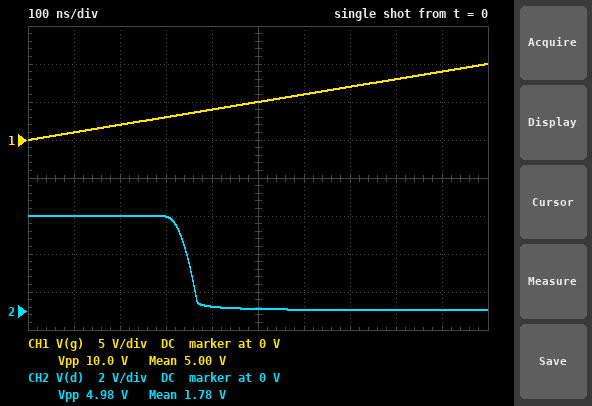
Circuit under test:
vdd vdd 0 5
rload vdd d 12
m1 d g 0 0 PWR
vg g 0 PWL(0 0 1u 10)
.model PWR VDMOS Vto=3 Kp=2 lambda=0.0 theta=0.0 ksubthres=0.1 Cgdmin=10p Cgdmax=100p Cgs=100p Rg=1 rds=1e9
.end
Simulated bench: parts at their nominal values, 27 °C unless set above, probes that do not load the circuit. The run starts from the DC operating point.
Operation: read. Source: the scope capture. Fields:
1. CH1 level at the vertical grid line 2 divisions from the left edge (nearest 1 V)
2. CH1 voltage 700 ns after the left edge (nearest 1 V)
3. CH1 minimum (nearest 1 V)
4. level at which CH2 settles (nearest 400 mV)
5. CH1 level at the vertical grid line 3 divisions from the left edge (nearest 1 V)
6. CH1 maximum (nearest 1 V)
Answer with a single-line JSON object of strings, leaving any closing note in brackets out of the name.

{"CH1 level at the vertical grid line 2 divisions from the left edge": "2 V", "CH1 voltage 700 ns after the left edge": "7 V", "CH1 minimum": "0 V", "level at which CH2 settles": "0 V", "CH1 level at the vertical grid line 3 divisions from the left edge": "3 V", "CH1 maximum": "10 V"}
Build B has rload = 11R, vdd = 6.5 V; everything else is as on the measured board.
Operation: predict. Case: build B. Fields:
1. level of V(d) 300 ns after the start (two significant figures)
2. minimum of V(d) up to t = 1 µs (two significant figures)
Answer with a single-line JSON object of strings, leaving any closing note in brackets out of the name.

{"level of V(d) 300 ns after the start": "6.5 V", "minimum of V(d) up to t = 1 µs": "42 mV"}
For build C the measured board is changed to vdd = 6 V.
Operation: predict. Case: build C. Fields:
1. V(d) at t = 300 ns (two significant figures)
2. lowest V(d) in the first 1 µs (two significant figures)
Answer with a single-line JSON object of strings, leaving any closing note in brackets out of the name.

{"V(d) at t = 300 ns": "6.0 V", "lowest V(d) in the first 1 µs": "36 mV"}
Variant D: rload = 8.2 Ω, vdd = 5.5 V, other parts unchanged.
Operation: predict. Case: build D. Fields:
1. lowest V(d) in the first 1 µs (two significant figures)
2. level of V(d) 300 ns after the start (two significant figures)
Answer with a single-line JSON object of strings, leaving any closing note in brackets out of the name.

{"lowest V(d) in the first 1 µs": "48 mV", "level of V(d) 300 ns after the start": "5.5 V"}
